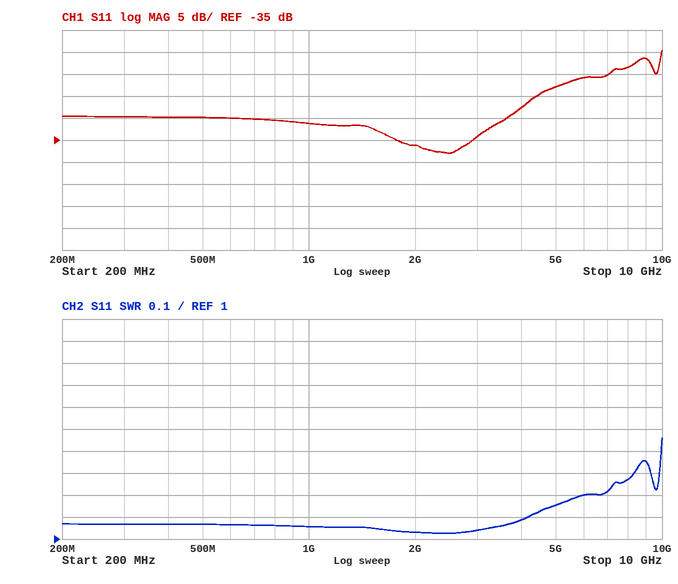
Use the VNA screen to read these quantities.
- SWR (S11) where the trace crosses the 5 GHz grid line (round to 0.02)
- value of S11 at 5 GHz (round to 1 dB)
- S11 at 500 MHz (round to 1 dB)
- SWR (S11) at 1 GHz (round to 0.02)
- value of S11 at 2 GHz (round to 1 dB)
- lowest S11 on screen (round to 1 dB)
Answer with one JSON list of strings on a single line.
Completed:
["1.16", "-23 dB", "-30 dB", "1.06", "-36 dB", "-38 dB"]
